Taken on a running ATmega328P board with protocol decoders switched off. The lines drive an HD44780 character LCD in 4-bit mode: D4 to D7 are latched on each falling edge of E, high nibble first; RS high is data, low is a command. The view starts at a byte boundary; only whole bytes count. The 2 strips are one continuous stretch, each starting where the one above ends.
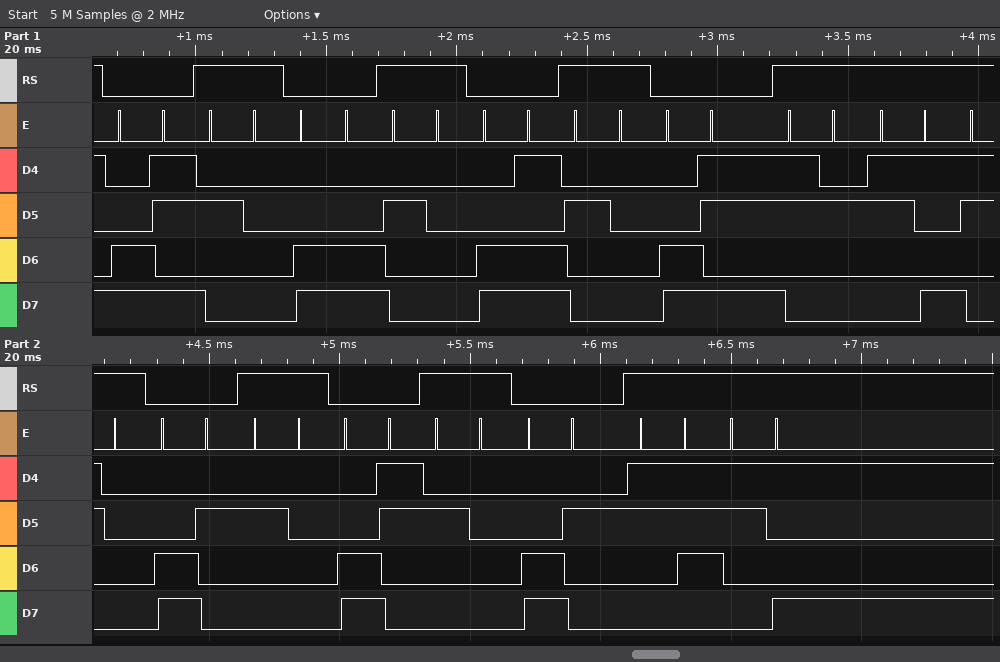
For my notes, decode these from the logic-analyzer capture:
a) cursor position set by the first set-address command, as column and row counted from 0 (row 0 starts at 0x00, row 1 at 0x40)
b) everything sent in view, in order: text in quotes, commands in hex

column 11, row 1
0xCB " " 0xCC " " 0xCD " " 0xCB "290" 0xC2 " " 0xC3 " " 0xC2 "79"
